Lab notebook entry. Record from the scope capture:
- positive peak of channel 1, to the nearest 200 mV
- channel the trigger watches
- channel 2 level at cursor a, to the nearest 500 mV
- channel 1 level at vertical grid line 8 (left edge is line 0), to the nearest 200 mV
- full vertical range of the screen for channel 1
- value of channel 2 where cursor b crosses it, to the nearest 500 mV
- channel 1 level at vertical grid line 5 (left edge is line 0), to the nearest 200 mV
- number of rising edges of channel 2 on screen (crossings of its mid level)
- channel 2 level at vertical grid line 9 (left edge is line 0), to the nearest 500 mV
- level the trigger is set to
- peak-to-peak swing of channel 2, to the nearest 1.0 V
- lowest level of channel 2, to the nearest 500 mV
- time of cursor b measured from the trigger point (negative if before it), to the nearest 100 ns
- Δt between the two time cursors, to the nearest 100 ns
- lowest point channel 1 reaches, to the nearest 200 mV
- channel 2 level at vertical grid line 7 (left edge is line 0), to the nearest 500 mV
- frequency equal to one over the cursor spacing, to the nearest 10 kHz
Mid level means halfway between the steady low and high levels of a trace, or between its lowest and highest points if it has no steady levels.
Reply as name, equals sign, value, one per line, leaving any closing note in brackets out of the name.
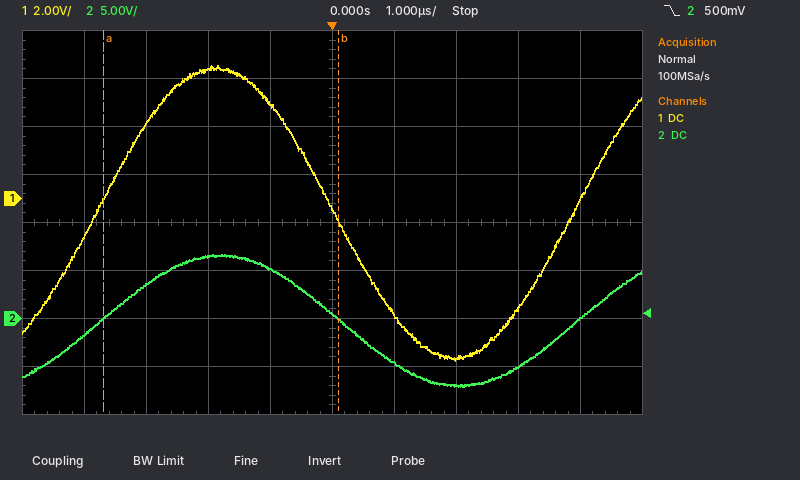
positive peak of channel 1, to the nearest 200 mV = 5.6 V
channel the trigger watches = channel 2
channel 2 level at cursor a, to the nearest 500 mV = 0.0 V
channel 1 level at vertical grid line 8 (left edge is line 0), to the nearest 200 mV = -4.6 V
full vertical range of the screen for channel 1 = 16 V
value of channel 2 where cursor b crosses it, to the nearest 500 mV = 0.0 V
channel 1 level at vertical grid line 5 (left edge is line 0), to the nearest 200 mV = -400 mV
number of rising edges of channel 2 on screen = 2
channel 2 level at vertical grid line 9 (left edge is line 0), to the nearest 500 mV = 0.0 V
level the trigger is set to = 500 mV
peak-to-peak swing of channel 2, to the nearest 1.0 V = 14.0 V
lowest level of channel 2, to the nearest 500 mV = -7.0 V
time of cursor b measured from the trigger point (negative if before it), to the nearest 100 ns = +100 ns
Δt between the two time cursors, to the nearest 100 ns = 3.8 µs
lowest point channel 1 reaches, to the nearest 200 mV = -6.8 V
channel 2 level at vertical grid line 7 (left edge is line 0), to the nearest 500 mV = -7.0 V
frequency equal to one over the cursor spacing, to the nearest 10 kHz = 260 kHz
